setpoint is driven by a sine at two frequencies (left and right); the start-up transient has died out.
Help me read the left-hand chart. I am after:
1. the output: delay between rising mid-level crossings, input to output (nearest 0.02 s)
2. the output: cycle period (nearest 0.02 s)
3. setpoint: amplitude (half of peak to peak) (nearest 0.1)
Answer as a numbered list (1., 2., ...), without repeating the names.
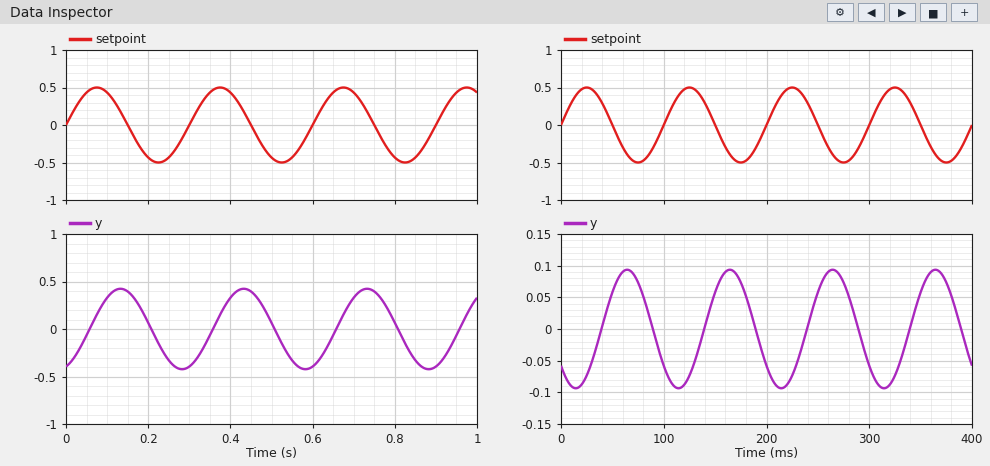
1. 0.06 s
2. 0.30 s
3. 0.5
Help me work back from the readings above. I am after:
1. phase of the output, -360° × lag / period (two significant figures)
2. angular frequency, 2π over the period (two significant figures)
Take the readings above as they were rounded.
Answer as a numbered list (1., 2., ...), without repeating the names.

1. -72°
2. 21 rad/s
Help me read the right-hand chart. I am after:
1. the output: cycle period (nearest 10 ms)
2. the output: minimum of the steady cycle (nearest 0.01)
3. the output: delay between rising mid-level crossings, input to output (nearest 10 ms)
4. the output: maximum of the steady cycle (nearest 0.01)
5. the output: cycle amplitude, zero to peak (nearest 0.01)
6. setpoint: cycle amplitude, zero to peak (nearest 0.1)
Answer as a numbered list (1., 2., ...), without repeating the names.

1. 100 ms
2. -0.09
3. 40 ms
4. 0.09
5. 0.09
6. 0.5
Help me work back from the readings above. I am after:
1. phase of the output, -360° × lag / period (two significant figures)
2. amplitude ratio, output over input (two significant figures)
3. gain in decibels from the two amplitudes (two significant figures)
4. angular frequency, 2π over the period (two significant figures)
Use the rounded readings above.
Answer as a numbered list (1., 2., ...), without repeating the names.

1. -140°
2. 0.18
3. -15 dB
4. 0.063 rad/ms
